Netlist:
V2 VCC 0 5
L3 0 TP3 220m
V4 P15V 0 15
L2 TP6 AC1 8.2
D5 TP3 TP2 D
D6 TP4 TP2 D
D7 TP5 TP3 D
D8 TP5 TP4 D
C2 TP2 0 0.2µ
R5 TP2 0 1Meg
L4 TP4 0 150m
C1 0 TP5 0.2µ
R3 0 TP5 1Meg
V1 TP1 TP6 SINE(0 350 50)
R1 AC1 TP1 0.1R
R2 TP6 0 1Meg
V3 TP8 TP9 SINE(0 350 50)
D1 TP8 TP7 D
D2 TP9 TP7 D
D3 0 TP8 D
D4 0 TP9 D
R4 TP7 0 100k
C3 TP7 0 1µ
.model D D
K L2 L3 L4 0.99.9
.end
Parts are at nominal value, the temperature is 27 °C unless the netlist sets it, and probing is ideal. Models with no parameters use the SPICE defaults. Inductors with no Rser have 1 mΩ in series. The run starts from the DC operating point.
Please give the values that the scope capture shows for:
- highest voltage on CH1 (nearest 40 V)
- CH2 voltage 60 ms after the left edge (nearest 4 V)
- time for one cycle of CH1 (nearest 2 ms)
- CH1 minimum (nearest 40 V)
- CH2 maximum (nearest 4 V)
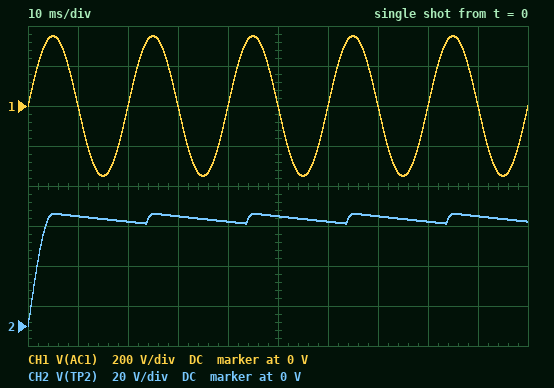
360 V
52 V
20 ms
-360 V
56 V
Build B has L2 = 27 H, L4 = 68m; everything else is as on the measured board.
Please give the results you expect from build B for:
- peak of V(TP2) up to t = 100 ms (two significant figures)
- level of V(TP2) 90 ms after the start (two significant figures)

31 V
30 V
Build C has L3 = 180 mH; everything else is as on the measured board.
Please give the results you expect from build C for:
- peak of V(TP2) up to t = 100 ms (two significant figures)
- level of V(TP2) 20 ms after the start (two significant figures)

51 V
47 V
